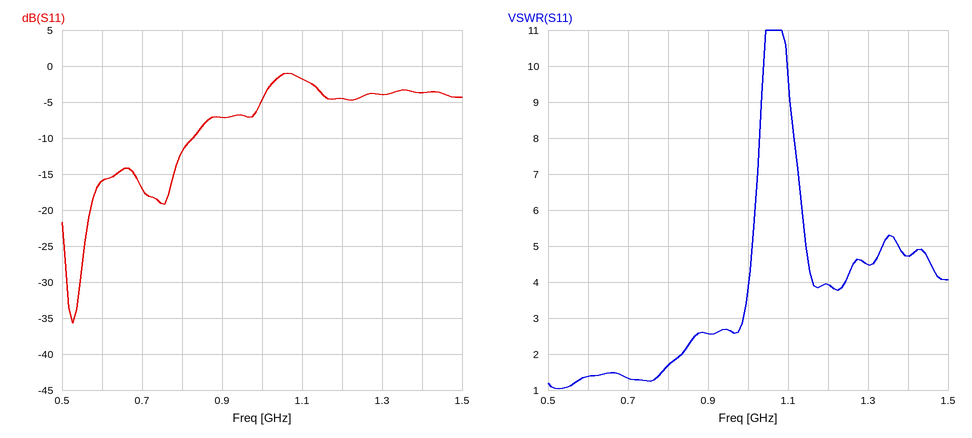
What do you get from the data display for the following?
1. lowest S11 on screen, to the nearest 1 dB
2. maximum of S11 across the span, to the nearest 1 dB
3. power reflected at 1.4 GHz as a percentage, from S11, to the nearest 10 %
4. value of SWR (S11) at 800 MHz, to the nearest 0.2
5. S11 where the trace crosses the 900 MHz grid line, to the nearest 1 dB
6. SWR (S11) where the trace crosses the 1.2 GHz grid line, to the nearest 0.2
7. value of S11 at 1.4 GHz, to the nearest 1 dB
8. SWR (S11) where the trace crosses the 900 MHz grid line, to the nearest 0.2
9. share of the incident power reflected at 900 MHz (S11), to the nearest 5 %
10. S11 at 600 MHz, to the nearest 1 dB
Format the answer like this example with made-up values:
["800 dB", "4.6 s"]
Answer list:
["-36 dB", "-1 dB", "40 %", "1.6", "-7 dB", "4.0", "-4 dB", "2.6", "20 %", "-16 dB"]
